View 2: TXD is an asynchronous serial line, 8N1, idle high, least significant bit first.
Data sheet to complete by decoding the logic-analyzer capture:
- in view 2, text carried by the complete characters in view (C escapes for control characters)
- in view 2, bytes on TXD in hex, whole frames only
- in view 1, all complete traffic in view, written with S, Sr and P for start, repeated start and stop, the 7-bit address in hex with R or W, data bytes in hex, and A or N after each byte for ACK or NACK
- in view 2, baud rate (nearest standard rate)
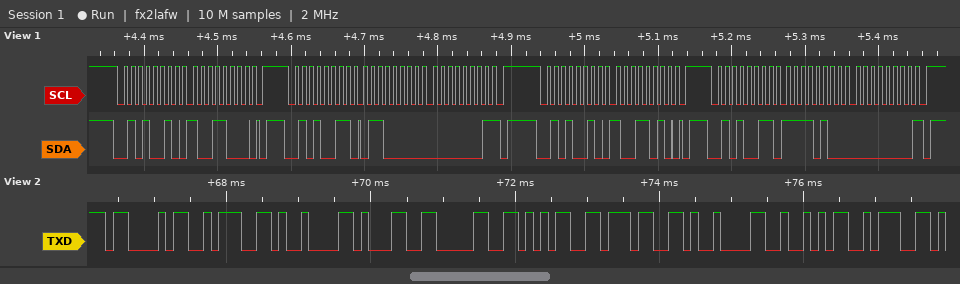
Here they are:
"C:\t1057\tR:"
43 3A 09 31 30 35 37 09 52 3A
S 29W A 98 A P S 29R A 60 A 01 N P S 29W A 9A A P S 29R A F4 A 00 N P
9600 baud
